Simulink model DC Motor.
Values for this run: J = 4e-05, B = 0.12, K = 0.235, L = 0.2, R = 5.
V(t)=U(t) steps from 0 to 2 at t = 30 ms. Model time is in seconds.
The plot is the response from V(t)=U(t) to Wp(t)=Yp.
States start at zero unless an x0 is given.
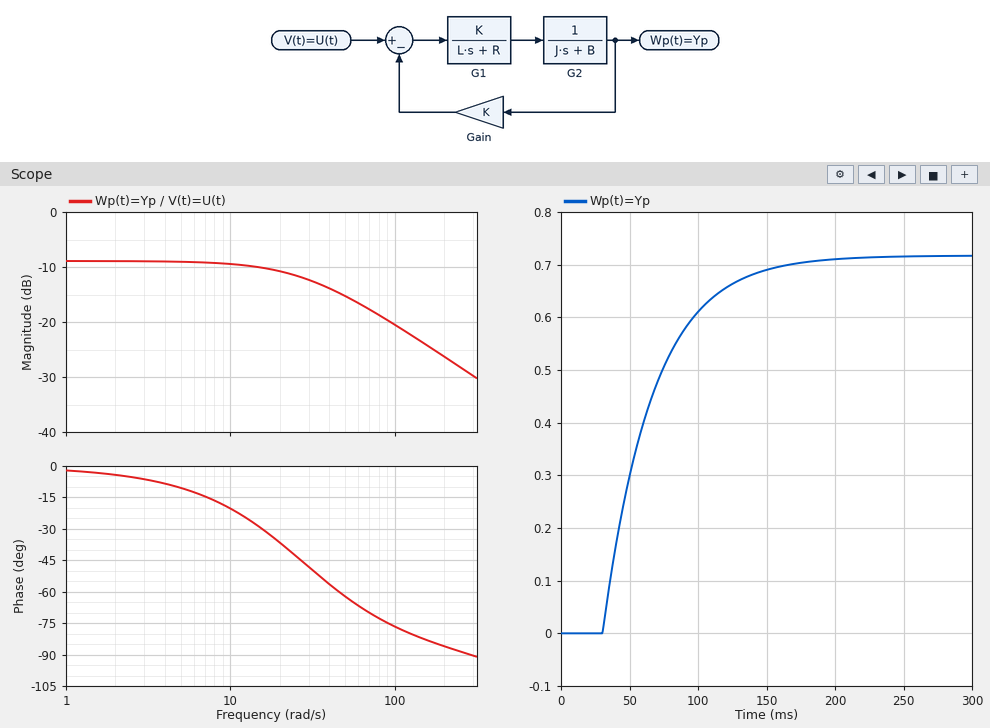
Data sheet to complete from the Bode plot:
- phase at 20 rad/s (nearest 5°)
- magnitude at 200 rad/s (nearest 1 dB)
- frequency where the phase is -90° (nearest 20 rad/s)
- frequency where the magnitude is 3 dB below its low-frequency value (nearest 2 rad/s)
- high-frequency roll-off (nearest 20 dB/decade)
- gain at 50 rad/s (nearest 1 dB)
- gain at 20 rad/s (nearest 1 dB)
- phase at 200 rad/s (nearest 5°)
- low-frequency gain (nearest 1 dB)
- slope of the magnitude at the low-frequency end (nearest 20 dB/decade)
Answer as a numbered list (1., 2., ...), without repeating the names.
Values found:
1. -35°
2. -26 dB
3. 280 rad/s
4. 28 rad/s
5. -20 dB/decade
6. -15 dB
7. -11 dB
8. -85°
9. -9 dB
10. 0 dB/decade
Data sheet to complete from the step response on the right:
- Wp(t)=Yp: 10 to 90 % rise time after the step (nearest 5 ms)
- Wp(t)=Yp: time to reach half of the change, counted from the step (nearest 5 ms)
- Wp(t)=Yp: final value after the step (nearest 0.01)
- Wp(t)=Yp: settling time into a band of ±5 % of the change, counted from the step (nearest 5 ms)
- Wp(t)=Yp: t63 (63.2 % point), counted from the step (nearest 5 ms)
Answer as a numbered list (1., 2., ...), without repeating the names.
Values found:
1. 80 ms
2. 25 ms
3. 0.72
4. 110 ms
5. 35 ms
